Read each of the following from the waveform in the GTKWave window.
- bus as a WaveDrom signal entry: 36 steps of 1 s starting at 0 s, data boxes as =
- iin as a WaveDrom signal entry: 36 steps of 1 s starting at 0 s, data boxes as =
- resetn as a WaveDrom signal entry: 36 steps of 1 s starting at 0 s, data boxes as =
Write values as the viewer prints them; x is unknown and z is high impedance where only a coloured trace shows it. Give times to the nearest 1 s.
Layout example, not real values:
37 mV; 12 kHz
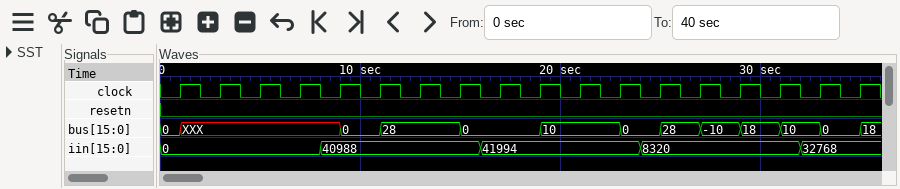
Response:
{name: 'bus', wave: '=x.......=.=...=...=...=.=.=.=.=.=.=', data: '0 0 28 0 10 0 28 -10 18 10 0 18'}; {name: 'iin', wave: '=.......=.......=.......=.......=...', data: '0 40988 41994 8320 32768'}; {name: 'resetn', wave: '0...................................'}
